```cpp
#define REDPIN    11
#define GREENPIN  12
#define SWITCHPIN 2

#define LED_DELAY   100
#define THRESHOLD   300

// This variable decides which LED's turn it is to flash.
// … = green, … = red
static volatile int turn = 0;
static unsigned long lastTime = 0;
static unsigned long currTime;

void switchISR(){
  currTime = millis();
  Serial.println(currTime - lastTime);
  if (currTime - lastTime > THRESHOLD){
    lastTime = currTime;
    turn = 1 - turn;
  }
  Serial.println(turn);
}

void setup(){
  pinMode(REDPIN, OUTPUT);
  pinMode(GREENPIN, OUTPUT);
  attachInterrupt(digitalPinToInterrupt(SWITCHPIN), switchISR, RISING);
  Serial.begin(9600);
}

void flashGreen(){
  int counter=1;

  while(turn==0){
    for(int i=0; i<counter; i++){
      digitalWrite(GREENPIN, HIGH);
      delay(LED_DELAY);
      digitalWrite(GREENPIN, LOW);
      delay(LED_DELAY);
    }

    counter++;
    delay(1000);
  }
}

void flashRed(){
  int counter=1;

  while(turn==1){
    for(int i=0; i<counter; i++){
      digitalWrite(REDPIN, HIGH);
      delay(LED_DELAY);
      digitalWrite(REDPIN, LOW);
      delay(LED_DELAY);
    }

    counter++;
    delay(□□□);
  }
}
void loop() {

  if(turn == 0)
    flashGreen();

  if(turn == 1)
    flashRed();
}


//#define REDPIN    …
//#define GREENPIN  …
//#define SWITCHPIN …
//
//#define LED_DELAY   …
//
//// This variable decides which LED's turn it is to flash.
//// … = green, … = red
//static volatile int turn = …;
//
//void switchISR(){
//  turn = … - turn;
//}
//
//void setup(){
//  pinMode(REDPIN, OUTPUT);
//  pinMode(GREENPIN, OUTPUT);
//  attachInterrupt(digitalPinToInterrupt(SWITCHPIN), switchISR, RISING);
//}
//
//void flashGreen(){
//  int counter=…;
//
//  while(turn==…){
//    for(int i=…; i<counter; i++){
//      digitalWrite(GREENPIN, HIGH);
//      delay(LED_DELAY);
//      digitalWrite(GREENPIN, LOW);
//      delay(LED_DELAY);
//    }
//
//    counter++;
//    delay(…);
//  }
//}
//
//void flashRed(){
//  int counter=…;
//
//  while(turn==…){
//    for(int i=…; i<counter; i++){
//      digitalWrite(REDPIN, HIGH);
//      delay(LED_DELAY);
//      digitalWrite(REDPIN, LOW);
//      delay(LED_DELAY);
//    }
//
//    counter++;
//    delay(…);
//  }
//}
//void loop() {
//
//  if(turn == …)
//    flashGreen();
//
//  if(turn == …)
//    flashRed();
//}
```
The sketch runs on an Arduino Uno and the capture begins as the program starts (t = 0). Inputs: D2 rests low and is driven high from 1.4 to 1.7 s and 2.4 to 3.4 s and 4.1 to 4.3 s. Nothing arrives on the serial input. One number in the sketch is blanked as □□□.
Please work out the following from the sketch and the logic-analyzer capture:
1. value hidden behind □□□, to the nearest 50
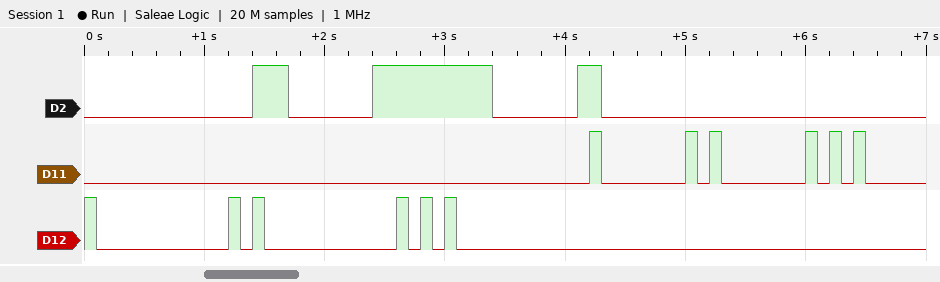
600
